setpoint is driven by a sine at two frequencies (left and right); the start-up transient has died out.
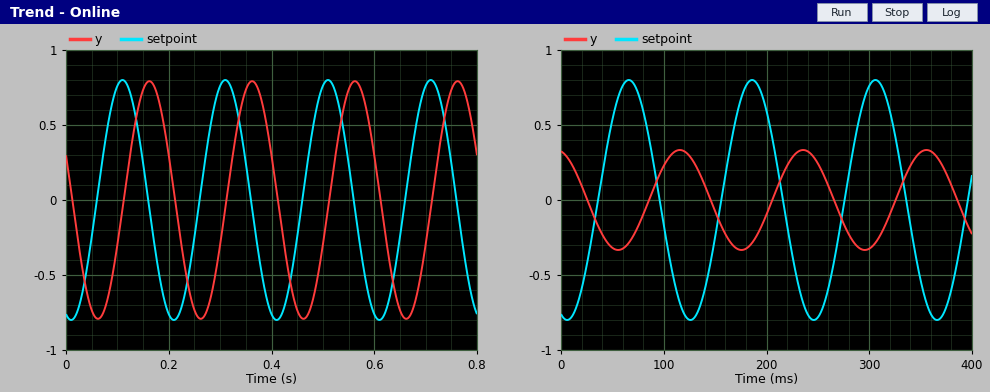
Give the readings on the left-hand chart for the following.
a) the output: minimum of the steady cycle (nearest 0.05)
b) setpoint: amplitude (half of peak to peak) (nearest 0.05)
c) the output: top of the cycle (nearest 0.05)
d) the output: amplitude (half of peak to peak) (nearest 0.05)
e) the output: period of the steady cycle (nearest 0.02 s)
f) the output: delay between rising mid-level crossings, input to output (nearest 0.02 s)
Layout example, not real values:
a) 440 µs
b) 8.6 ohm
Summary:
a) -0.80
b) 0.80
c) 0.80
d) 0.80
e) 0.20 s
f) 0.06 s
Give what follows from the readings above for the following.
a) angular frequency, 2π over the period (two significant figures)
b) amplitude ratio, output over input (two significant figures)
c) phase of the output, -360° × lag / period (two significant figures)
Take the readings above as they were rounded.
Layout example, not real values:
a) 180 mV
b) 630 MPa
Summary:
a) 31 rad/s
b) 1.0
c) -110°
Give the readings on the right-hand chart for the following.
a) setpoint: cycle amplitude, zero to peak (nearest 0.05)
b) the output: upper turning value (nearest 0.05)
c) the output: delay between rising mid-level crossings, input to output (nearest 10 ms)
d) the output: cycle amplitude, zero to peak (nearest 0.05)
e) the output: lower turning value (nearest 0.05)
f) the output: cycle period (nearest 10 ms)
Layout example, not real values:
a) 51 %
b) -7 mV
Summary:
a) 0.80
b) 0.35
c) 50 ms
d) 0.35
e) -0.35
f) 120 ms
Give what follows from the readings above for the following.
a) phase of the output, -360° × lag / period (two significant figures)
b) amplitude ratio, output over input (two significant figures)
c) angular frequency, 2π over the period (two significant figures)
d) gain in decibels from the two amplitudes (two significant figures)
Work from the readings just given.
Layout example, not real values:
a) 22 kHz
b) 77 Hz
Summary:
a) -150°
b) 0.44
c) 0.052 rad/ms
d) -7.2 dB
